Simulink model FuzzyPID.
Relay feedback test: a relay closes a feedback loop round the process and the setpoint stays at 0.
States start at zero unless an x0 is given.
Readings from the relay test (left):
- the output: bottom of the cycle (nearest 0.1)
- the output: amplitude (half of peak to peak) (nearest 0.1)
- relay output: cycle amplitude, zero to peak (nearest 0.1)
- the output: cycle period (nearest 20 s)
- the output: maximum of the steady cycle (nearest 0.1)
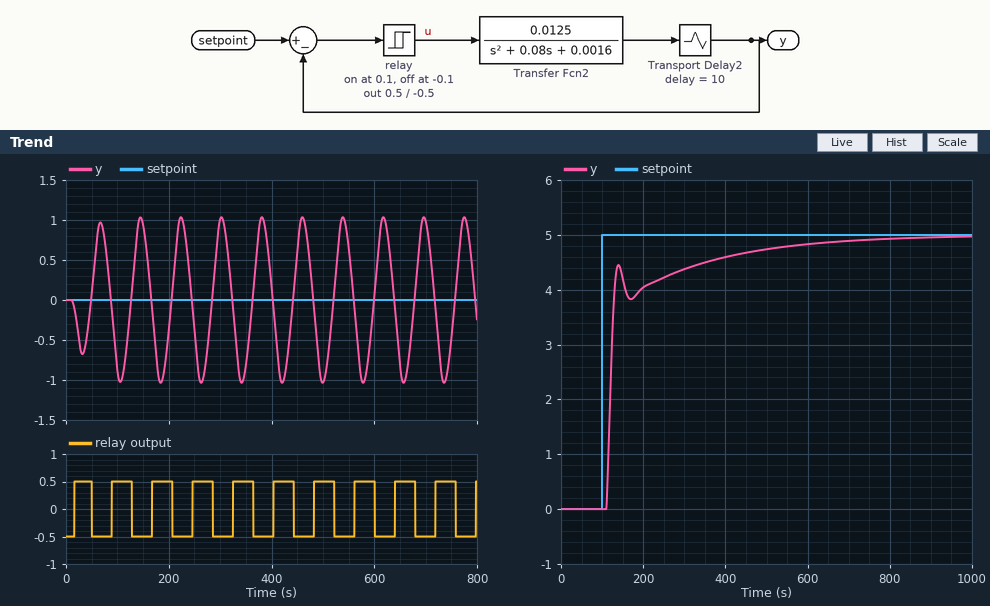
-1.0
1.0
0.5
80 s
1.0
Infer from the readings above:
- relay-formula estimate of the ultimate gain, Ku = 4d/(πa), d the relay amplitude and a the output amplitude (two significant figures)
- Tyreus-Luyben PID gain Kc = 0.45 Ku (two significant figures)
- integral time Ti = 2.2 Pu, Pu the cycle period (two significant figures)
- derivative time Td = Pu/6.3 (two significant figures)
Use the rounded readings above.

0.64
0.29
180 s
13 s
